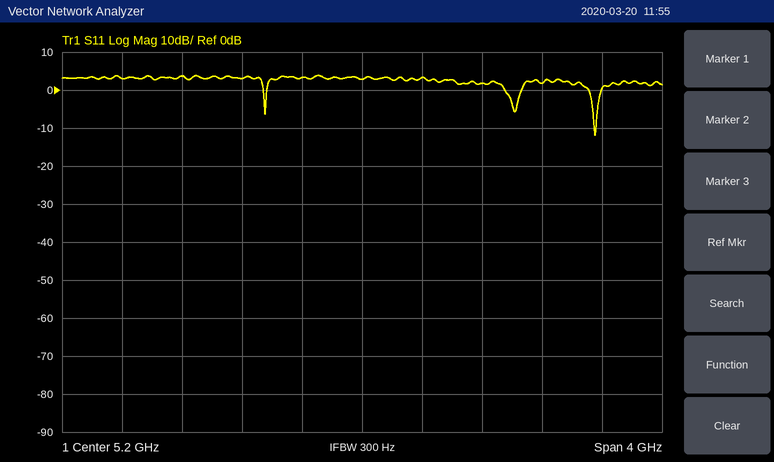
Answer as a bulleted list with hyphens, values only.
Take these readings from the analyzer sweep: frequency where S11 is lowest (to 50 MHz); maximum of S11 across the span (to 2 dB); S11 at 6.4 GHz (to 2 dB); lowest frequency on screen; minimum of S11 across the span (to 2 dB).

- 6.75 GHz
- 4 dB
- 2 dB
- 3.2 GHz
- -12 dB
